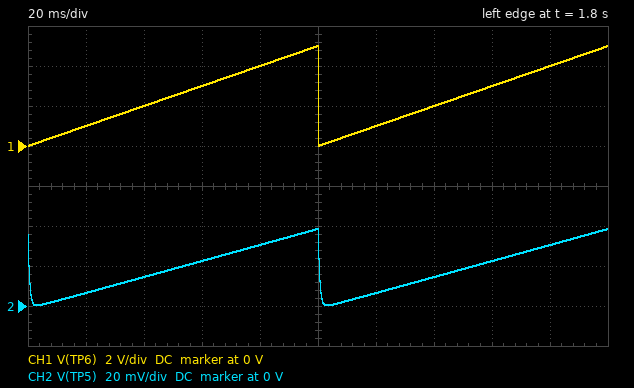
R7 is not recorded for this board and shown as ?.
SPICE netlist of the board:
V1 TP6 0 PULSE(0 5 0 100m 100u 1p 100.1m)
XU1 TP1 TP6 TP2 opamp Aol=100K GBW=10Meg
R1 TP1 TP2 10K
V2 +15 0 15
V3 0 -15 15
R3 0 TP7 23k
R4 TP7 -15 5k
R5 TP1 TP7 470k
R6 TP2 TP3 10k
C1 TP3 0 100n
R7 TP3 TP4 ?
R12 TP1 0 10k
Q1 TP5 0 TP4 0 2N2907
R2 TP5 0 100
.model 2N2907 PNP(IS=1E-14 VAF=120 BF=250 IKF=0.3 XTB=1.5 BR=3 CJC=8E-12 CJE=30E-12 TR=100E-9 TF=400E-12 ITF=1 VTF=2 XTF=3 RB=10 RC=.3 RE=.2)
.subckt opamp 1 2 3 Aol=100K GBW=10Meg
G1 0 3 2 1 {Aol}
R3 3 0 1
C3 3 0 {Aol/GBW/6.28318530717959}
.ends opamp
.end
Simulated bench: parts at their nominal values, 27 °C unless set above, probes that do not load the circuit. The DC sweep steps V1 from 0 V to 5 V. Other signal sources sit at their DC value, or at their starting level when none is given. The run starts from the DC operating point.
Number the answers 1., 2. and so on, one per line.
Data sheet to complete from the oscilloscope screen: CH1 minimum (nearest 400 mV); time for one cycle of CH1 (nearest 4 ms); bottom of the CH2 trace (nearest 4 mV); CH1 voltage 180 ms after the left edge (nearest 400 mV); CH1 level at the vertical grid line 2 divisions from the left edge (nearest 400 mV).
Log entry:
1. 0 V
2. 100 ms
3. 0 V
4. 4.0 V
5. 2.0 V
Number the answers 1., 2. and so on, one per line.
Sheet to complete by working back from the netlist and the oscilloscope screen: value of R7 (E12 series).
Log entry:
1. 15 kΩ
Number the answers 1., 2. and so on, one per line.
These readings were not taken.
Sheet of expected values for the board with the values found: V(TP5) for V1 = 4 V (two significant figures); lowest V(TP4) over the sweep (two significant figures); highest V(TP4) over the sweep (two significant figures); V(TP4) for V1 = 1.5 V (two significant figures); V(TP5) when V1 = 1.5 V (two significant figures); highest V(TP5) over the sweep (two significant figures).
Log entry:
1. 31 mV
2. 260 mV
3. 630 mV
4. 600 mV
5. 11 mV
6. 39 mV
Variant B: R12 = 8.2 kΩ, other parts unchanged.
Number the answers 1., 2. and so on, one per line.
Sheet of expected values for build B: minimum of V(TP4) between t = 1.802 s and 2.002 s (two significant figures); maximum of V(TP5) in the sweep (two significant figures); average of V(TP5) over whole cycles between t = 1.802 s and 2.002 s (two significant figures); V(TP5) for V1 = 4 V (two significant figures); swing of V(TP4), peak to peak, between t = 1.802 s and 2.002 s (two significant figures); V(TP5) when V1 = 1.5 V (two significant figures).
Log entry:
1. 510 mV
2. 43 mV
3. 21 mV
4. 34 mV
5. 120 mV
6. 12 mV
